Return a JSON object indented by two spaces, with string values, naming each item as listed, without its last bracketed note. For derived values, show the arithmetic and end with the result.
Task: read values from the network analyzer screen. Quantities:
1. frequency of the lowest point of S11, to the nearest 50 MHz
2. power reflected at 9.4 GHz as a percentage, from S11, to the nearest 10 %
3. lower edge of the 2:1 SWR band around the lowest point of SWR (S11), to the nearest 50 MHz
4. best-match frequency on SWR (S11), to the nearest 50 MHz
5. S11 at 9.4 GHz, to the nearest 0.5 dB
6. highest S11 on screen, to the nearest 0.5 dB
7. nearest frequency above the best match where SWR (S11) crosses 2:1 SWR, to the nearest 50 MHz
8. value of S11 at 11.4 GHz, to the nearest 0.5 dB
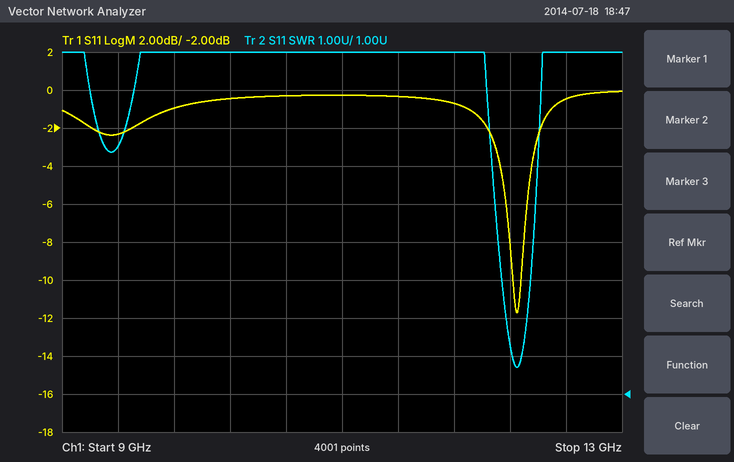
{
  "frequency of the lowest point of S11, to the nearest 50 MHz": "12.25 GHz",
  "power reflected at 9.4 GHz as a percentage, from S11, to the nearest 10 %": "10^(-2.5/10) ≈ 56.2 %, so 60 % to the nearest 10 %",
  "lower edge of the 2:1 SWR band around the lowest point of SWR (S11), to the nearest 50 MHz": "12.20 GHz",
  "best-match frequency on SWR (S11), to the nearest 50 MHz": "12.25 GHz",
  "S11 at 9.4 GHz, to the nearest 0.5 dB": "-2.5 dB",
  "highest S11 on screen, to the nearest 0.5 dB": "0.0 dB",
  "nearest frequency above the best match where SWR (S11) crosses 2:1 SWR, to the nearest 50 MHz": "12.30 GHz",
  "value of S11 at 11.4 GHz, to the nearest 0.5 dB": "-0.5 dB"
}
